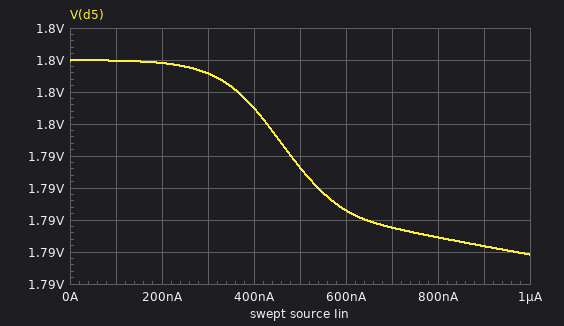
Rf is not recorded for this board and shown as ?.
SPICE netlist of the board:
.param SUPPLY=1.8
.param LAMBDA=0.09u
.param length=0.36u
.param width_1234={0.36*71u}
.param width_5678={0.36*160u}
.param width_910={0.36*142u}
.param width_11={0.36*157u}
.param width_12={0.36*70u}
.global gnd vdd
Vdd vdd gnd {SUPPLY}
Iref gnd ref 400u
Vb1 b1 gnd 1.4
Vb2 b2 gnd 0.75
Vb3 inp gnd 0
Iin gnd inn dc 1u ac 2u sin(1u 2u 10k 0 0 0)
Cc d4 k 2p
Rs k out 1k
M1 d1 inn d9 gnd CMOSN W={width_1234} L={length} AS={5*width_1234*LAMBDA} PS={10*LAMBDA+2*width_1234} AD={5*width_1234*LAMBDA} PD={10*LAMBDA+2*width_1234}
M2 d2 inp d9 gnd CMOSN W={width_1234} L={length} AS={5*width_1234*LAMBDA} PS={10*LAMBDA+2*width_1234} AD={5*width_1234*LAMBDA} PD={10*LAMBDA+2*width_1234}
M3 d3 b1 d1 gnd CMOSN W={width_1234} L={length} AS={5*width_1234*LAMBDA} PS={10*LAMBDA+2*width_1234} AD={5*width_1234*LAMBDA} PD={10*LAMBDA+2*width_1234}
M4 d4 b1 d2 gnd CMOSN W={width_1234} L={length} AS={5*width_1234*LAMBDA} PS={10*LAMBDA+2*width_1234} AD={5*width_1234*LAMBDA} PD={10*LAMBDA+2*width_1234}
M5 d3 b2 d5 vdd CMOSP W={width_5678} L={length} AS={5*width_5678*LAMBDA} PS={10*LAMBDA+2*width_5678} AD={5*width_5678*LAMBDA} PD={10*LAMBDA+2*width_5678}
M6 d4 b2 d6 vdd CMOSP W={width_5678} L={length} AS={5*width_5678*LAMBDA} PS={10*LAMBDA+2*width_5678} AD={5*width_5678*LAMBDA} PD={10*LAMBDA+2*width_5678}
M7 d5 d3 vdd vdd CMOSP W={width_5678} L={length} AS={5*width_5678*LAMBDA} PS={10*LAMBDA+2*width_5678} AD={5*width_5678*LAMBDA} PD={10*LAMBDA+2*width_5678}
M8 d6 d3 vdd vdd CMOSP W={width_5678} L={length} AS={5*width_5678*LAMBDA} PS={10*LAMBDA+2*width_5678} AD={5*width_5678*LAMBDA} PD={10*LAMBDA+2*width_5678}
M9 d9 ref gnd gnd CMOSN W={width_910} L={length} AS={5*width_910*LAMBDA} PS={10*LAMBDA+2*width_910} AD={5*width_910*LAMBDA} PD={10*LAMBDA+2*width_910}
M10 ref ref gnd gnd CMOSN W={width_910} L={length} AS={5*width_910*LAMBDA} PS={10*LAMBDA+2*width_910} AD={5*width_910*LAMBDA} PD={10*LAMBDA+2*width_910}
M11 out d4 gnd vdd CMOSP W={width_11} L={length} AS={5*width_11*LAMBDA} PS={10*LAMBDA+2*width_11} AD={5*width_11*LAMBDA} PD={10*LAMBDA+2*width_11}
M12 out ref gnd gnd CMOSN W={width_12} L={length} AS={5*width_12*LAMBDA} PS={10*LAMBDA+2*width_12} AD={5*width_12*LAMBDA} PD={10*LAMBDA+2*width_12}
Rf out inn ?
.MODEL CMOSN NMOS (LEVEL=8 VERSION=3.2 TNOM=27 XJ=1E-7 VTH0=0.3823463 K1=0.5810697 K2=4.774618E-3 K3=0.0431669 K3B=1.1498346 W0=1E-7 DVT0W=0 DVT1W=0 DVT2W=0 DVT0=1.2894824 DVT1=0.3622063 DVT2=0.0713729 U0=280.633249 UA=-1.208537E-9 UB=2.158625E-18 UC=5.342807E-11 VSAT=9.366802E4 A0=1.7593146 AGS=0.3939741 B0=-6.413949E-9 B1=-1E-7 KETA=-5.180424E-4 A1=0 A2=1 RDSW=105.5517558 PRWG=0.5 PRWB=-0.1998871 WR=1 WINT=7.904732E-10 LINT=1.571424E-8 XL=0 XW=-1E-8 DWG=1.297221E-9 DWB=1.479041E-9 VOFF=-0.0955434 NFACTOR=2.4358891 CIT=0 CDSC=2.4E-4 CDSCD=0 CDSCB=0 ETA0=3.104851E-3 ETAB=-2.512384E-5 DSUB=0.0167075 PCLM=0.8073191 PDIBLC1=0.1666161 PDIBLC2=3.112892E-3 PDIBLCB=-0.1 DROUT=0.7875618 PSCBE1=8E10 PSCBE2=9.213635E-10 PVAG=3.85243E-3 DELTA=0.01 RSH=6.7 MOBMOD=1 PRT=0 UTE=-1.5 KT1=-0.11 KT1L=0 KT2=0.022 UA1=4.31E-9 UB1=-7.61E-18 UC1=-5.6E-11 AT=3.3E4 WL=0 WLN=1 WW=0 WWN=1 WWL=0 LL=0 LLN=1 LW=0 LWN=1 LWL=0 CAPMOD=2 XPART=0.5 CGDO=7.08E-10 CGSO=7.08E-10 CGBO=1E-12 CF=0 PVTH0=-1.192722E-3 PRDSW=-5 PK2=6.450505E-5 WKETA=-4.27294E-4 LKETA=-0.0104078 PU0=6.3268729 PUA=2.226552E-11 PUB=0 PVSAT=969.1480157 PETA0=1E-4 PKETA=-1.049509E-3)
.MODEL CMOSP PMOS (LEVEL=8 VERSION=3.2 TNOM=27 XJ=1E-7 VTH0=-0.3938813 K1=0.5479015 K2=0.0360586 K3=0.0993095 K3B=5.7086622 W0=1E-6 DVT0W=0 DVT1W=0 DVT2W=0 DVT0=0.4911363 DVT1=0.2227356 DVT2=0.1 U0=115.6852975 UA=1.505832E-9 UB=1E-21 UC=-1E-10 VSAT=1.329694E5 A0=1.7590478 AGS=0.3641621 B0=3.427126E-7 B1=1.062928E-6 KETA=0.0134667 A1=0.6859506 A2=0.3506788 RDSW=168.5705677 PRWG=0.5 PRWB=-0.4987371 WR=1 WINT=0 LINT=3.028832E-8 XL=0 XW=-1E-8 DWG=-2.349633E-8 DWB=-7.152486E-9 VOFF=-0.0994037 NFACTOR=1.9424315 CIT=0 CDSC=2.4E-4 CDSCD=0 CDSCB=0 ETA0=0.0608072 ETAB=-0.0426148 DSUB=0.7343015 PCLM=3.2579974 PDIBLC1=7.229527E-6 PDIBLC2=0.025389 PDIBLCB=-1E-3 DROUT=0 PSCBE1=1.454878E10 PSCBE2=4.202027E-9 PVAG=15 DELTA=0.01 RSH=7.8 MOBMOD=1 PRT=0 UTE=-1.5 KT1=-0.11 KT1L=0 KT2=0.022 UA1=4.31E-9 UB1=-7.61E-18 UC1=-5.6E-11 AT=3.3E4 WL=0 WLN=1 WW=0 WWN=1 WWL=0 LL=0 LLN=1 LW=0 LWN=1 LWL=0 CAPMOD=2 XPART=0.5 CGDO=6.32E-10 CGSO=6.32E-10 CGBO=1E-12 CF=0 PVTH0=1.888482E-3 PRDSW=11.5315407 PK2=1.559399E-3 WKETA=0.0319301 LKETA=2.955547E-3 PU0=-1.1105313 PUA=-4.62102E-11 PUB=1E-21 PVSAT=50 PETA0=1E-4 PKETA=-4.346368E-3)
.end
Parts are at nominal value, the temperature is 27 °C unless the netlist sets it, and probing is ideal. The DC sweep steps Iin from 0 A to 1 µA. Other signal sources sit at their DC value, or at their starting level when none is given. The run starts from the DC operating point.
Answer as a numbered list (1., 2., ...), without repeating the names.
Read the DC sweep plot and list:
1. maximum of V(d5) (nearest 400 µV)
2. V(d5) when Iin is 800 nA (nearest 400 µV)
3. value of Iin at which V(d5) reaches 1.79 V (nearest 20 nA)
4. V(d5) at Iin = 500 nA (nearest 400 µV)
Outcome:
1. 1.8000 V
2. 1.7888 V
3. 480 nA
4. 1.7932 V
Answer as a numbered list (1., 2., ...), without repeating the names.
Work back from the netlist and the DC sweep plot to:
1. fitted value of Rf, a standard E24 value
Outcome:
1. 1.1 MΩ
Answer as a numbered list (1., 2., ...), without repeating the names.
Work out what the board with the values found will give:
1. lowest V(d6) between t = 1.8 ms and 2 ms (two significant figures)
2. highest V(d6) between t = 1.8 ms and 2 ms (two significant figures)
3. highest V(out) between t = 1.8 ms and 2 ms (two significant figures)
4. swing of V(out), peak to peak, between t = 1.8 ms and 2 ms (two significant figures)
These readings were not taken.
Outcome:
1. 1.8 V
2. 1.8 V
3. 1.7 mV
4. 2.3 mV
